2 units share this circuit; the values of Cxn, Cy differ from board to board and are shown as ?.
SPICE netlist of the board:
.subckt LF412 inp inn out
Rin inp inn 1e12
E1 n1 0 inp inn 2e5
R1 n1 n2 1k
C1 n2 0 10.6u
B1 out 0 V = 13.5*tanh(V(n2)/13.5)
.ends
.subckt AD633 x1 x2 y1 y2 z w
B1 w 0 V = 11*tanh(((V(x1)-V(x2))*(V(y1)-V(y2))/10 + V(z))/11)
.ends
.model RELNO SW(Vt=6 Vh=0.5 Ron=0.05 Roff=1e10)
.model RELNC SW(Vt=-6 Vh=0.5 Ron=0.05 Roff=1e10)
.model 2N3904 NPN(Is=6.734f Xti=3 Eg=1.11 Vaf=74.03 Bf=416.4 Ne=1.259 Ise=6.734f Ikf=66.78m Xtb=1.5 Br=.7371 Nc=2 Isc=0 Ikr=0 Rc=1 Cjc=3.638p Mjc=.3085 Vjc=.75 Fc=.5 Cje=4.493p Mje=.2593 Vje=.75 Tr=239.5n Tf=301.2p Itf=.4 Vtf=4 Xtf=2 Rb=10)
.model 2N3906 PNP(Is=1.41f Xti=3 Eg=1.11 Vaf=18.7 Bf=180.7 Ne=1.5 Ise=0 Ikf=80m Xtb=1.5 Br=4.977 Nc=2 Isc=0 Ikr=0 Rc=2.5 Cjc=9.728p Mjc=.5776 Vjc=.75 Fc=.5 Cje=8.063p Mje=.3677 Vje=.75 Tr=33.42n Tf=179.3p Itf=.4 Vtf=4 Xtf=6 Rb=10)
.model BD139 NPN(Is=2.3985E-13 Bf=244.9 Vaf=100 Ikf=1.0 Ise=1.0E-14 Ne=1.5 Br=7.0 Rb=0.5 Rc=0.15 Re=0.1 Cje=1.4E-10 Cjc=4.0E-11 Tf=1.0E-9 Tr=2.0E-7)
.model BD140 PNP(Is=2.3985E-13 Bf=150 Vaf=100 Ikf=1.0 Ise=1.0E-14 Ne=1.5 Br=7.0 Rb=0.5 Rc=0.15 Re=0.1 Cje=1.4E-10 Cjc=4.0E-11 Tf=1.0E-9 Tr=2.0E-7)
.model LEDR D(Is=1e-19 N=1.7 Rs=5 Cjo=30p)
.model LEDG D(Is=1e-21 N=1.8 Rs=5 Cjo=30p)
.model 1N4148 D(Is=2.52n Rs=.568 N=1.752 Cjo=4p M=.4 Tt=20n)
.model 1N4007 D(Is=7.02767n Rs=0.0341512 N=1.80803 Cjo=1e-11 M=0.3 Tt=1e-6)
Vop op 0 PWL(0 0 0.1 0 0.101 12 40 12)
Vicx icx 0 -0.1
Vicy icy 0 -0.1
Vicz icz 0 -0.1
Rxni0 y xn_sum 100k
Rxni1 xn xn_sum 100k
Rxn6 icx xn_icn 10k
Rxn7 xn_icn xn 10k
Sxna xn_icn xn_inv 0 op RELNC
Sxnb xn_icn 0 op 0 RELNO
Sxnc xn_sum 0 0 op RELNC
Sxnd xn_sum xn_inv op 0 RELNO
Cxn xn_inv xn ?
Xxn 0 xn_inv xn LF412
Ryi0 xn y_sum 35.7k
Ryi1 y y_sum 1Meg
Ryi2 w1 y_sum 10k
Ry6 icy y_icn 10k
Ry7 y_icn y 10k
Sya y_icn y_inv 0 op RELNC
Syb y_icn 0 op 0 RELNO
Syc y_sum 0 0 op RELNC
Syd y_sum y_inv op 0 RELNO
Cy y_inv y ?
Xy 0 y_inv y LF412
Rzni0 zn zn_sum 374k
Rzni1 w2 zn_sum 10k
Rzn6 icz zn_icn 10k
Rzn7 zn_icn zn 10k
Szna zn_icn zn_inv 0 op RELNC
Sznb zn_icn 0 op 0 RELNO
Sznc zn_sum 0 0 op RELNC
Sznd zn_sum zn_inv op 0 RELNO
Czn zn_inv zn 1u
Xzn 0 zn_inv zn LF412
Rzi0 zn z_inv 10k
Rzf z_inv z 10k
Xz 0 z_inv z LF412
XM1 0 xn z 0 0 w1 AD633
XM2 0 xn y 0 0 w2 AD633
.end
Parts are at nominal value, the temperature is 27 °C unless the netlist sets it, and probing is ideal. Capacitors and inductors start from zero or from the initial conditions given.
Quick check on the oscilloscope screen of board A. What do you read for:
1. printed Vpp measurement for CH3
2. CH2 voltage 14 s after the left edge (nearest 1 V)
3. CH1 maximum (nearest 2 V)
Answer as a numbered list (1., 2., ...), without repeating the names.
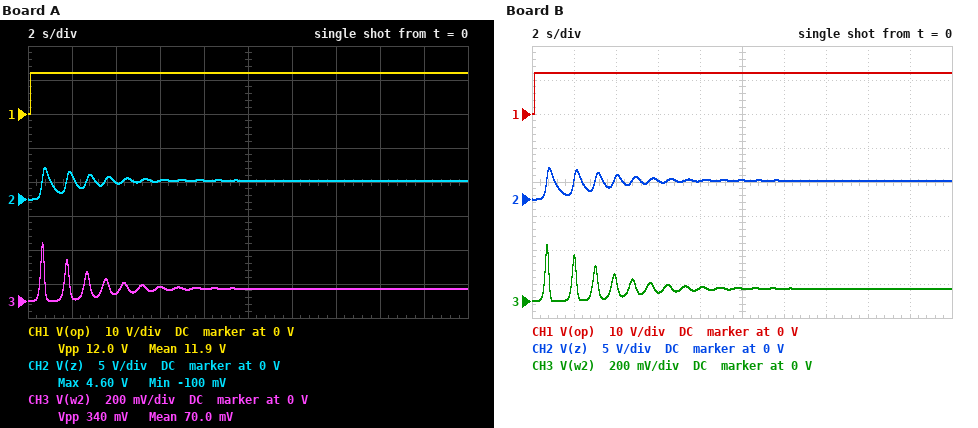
1. 340 mV
2. 3 V
3. 12 V
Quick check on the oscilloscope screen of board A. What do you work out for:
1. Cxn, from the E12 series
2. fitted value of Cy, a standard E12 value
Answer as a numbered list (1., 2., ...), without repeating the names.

1. 560 nF
2. 2.2 µF
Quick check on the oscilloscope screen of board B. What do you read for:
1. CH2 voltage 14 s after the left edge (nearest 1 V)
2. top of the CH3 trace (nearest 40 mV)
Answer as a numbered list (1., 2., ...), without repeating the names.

1. 3 V
2. 320 mV
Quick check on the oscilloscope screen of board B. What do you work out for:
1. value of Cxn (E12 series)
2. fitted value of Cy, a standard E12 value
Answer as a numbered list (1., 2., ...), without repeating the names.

1. 680 nF
2. 2.2 µF
